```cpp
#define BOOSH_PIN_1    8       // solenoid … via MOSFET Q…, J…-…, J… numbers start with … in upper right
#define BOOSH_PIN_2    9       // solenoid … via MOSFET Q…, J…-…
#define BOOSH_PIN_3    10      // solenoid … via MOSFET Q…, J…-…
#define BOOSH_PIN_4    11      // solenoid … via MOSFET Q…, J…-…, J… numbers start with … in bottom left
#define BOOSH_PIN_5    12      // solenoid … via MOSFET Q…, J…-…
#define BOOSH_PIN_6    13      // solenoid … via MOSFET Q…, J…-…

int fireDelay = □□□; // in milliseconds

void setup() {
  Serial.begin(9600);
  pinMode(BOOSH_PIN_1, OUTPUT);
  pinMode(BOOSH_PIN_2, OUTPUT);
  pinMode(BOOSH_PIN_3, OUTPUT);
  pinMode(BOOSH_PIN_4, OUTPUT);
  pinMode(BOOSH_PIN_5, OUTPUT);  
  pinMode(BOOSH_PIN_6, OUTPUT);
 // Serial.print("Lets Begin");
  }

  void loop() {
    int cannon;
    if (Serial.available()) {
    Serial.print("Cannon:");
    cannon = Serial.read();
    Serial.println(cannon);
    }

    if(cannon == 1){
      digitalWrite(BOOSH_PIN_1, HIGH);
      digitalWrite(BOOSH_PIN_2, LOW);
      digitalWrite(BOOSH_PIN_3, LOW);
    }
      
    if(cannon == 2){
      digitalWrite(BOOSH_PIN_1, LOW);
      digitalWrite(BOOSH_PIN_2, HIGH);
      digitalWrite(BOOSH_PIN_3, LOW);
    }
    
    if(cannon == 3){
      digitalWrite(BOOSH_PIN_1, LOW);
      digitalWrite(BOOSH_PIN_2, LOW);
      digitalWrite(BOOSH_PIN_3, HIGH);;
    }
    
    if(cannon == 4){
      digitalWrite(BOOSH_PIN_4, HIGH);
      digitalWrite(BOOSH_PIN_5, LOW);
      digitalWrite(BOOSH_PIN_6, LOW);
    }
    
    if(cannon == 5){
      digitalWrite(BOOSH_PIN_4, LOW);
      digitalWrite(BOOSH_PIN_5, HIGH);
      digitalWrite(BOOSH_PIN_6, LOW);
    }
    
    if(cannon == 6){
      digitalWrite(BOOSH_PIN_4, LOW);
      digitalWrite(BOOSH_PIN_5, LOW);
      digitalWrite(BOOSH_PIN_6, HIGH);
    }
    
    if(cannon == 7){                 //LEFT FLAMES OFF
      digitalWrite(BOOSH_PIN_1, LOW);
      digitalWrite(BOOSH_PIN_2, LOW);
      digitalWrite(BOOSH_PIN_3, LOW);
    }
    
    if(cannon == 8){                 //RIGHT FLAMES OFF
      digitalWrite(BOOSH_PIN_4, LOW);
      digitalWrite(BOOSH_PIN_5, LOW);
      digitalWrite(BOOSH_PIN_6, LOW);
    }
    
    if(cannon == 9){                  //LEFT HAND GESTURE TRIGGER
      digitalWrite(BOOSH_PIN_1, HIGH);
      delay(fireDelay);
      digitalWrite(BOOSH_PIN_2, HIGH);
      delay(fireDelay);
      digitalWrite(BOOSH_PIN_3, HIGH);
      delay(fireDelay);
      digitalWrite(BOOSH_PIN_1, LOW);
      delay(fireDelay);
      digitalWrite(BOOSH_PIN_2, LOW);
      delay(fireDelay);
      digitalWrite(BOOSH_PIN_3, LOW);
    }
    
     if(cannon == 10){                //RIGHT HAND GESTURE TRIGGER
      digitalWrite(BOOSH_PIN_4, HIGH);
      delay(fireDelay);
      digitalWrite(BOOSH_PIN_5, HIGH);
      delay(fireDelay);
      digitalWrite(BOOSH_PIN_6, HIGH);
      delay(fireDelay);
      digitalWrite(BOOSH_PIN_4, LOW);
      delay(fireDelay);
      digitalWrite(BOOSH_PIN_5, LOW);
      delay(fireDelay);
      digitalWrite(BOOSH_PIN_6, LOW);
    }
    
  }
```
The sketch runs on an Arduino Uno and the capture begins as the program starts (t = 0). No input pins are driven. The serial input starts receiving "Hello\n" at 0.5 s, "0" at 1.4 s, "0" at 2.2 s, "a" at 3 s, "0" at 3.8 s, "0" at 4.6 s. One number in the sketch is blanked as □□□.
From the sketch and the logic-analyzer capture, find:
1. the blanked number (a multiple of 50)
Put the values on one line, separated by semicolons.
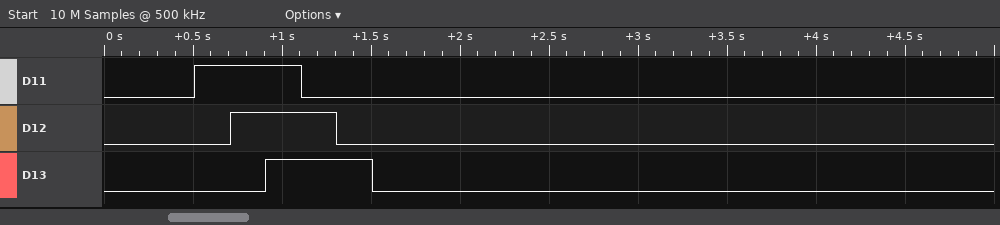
200
